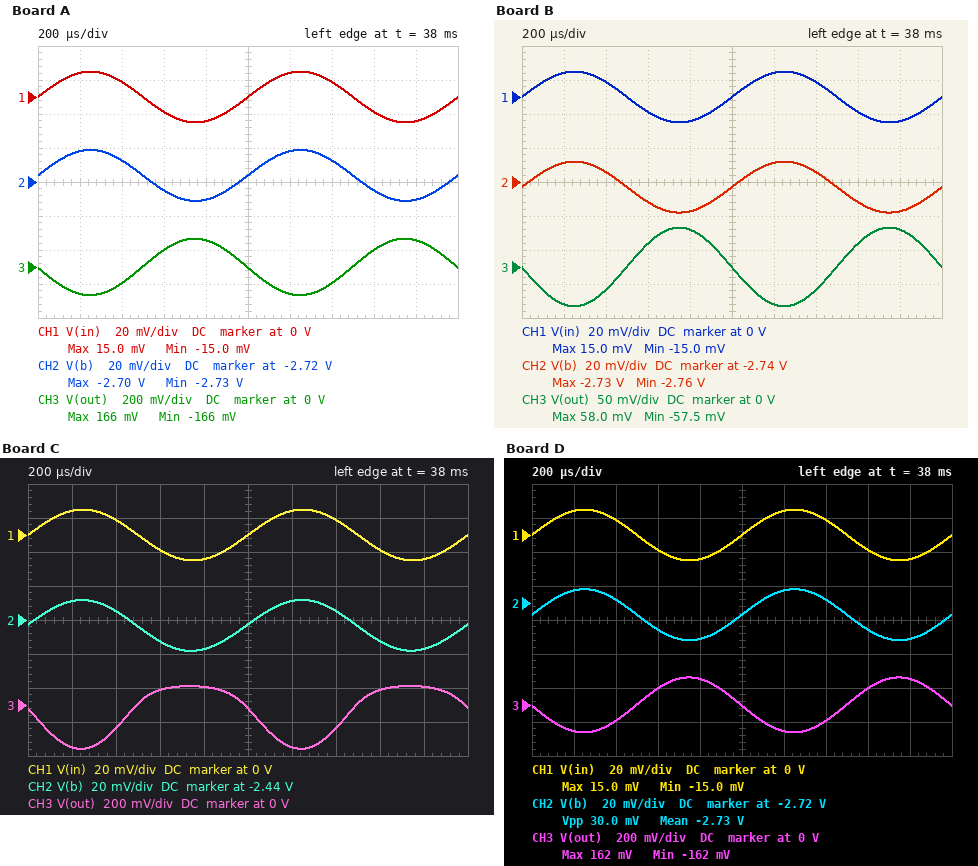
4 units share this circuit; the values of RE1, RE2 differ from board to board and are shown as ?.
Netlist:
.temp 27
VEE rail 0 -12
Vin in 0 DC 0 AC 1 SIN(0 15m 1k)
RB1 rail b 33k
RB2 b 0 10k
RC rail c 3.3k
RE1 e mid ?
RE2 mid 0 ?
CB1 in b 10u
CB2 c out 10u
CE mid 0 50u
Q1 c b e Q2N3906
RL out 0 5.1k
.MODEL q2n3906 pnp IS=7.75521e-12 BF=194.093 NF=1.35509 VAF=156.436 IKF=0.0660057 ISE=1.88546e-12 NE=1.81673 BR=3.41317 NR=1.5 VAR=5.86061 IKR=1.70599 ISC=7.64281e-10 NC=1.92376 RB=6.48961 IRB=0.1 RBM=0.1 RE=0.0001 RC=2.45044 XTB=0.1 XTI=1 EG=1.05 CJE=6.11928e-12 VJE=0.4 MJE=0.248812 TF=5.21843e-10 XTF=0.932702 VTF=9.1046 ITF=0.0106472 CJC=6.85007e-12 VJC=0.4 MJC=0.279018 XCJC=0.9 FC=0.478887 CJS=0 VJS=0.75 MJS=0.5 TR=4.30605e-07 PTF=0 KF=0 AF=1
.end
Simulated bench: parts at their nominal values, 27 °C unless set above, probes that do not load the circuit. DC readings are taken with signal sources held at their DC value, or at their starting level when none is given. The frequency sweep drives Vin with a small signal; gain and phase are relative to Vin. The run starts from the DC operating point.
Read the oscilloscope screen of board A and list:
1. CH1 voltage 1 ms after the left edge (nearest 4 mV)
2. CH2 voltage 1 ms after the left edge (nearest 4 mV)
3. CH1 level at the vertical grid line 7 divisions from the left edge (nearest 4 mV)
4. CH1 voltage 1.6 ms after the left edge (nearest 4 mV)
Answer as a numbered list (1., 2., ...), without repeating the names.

1. 0 V
2. -2.716 V
3. 8 mV
4. -8 mV
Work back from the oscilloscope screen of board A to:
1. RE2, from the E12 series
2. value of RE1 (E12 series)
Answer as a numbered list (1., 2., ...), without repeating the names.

1. 1.5 kΩ
2. 150 Ω
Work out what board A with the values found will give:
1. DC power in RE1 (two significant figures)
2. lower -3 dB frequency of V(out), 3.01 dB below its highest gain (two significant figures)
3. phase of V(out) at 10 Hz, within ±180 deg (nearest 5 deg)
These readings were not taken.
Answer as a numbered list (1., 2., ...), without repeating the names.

1. 230 µW
2. 21 Hz
3. -105 deg
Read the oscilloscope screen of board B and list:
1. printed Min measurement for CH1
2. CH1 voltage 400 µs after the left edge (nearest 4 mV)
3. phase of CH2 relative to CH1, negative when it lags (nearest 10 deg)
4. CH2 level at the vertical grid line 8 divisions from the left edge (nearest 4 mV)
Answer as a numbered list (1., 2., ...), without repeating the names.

1. -15.0 mV
2. 8 mV
3. 0 deg
4. -2.752 V
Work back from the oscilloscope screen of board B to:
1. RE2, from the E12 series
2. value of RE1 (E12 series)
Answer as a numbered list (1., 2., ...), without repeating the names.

1. 2.2 kΩ
2. 470 Ω
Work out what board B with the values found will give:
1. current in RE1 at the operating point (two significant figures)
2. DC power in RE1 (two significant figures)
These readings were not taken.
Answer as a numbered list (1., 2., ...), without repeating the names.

1. 780 µA
2. 290 µW
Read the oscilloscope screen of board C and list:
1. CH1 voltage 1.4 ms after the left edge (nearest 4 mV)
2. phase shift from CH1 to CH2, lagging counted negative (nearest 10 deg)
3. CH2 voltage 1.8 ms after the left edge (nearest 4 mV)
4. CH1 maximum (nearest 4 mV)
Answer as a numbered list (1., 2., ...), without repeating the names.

1. 8 mV
2. 0 deg
3. -2.456 V
4. 16 mV
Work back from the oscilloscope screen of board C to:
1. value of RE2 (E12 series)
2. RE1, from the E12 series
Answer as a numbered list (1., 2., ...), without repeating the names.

1. 470 Ω
2. 100 Ω
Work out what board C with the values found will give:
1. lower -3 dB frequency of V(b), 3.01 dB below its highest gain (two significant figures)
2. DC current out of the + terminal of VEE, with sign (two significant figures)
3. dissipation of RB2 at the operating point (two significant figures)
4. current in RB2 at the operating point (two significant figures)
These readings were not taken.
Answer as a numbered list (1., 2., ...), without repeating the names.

1. 80 Hz
2. -3.3 mA
3. 600 µW
4. 250 µA
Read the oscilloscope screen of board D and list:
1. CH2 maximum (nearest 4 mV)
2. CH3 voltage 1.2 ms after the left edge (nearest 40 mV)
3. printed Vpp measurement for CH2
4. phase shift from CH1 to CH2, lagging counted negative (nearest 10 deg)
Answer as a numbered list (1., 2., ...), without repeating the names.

1. -2.712 V
2. -160 mV
3. 30.0 mV
4. 0 deg
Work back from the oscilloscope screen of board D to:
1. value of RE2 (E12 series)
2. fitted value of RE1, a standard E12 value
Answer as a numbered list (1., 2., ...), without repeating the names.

1. 1.8 kΩ
2. 150 Ω
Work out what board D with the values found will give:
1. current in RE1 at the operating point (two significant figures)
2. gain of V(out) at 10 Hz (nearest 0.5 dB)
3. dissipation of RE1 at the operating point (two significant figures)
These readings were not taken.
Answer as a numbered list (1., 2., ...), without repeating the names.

1. 1.1 mA
2. 13.5 dB
3. 170 µW
